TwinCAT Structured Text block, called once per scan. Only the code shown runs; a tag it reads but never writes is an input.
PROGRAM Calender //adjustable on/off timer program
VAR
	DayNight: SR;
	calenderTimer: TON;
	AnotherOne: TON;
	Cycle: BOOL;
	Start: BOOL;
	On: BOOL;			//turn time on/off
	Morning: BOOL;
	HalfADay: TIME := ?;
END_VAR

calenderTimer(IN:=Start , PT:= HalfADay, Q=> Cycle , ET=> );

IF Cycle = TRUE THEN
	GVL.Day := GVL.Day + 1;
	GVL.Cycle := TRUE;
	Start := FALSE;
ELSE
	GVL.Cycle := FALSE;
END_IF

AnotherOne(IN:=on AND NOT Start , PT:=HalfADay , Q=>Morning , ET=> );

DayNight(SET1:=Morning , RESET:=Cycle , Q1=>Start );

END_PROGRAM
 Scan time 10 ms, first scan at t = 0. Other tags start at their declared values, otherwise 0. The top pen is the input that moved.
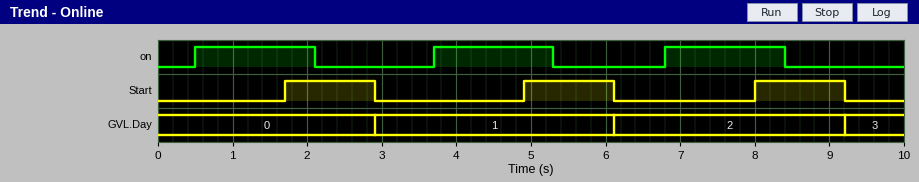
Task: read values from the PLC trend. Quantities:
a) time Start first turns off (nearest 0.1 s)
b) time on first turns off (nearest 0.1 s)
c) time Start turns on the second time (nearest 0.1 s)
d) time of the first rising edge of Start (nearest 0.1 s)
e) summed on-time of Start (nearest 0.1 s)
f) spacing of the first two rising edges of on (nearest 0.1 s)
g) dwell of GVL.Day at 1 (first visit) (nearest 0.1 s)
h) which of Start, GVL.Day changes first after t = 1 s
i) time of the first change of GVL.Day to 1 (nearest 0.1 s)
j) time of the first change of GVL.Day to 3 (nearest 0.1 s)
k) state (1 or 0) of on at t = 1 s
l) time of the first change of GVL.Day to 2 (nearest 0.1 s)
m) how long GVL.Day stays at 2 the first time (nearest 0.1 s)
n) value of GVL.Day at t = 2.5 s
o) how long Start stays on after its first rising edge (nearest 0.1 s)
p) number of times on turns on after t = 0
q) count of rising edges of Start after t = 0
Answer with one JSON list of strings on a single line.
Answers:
["2.9 s", "2.1 s", "4.9 s", "1.7 s", "3.6 s", "3.2 s", "3.2 s", "Start", "2.9 s", "9.2 s", "1", "6.1 s", "3.1 s", "0", "1.2 s", "3", "3"]
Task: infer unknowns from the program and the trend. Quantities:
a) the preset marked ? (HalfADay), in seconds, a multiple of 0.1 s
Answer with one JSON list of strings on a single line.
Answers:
["1.2 s"]
